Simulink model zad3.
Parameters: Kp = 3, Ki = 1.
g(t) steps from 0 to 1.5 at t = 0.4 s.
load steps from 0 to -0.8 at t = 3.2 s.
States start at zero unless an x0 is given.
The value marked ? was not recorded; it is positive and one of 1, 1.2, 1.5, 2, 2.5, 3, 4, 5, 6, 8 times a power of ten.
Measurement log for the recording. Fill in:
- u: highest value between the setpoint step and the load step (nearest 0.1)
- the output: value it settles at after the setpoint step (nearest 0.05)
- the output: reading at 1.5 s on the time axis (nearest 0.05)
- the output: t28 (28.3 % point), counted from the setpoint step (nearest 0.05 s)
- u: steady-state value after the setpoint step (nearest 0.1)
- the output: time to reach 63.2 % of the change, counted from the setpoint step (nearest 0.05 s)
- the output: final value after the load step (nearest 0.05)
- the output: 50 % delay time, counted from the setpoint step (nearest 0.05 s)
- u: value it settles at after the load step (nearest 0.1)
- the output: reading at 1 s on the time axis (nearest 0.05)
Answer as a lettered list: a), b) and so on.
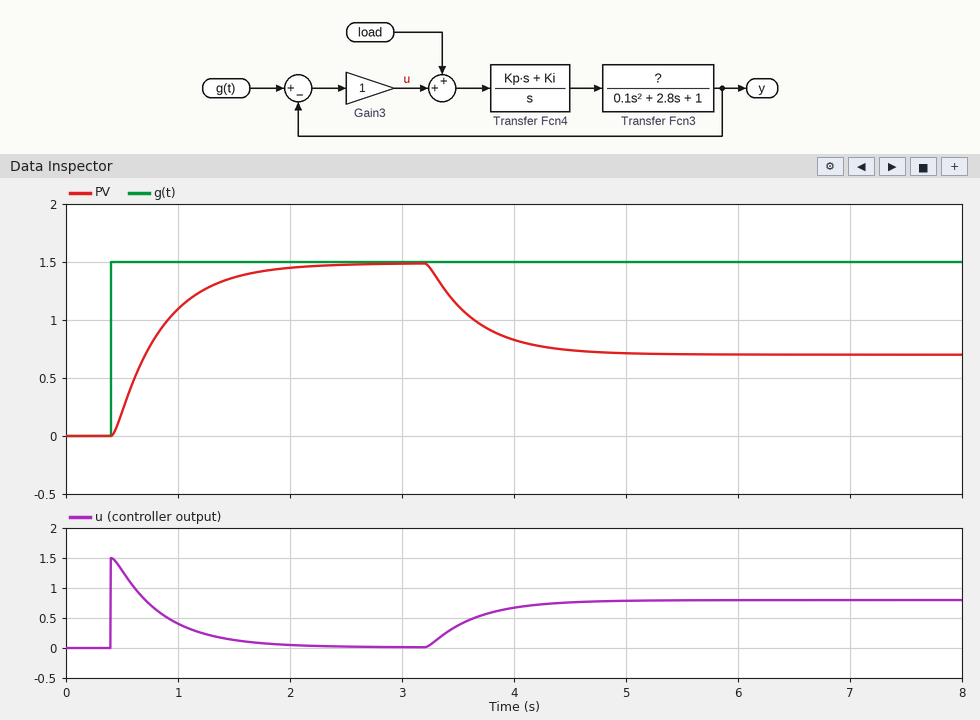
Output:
a) 1.5
b) 1.50
c) 1.35
d) 0.20 s
e) 0.0
f) 0.45 s
g) 0.70
h) 0.35 s
i) 0.8
j) 1.10
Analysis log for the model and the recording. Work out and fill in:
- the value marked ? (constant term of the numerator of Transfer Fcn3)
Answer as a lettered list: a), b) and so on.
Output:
a) 2
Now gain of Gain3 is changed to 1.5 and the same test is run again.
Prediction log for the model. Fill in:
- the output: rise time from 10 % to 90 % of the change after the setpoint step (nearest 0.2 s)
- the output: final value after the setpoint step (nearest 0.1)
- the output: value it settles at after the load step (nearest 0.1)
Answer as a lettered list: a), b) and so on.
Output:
a) 0.6 s
b) 1.5
c) 1.0
